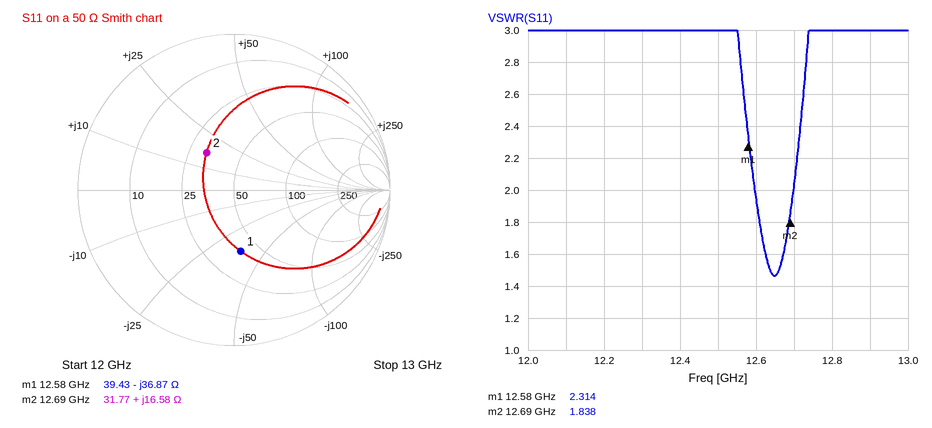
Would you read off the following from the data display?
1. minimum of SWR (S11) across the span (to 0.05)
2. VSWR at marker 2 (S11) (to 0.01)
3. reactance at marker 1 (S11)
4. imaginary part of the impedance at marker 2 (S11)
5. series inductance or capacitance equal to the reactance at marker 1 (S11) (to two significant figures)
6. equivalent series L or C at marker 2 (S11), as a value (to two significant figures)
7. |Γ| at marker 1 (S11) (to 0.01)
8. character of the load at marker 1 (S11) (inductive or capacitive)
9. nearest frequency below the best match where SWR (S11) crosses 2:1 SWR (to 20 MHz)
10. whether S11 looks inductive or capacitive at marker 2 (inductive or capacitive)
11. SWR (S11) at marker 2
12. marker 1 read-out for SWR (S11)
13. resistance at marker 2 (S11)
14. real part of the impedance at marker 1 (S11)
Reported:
1.45
1.84
-36.87 Ω
+16.58 Ω
340 fF
210 pH
0.40
capacitive
12.60 GHz
inductive
1.838
2.314
31.77 Ω
39.43 Ω
